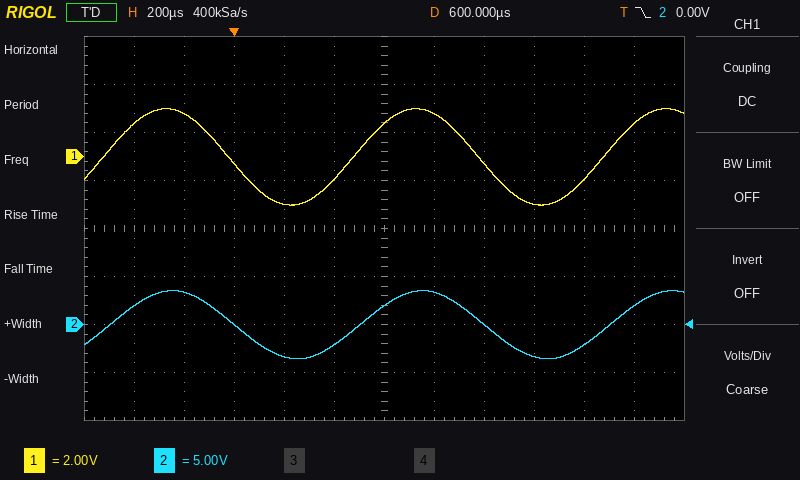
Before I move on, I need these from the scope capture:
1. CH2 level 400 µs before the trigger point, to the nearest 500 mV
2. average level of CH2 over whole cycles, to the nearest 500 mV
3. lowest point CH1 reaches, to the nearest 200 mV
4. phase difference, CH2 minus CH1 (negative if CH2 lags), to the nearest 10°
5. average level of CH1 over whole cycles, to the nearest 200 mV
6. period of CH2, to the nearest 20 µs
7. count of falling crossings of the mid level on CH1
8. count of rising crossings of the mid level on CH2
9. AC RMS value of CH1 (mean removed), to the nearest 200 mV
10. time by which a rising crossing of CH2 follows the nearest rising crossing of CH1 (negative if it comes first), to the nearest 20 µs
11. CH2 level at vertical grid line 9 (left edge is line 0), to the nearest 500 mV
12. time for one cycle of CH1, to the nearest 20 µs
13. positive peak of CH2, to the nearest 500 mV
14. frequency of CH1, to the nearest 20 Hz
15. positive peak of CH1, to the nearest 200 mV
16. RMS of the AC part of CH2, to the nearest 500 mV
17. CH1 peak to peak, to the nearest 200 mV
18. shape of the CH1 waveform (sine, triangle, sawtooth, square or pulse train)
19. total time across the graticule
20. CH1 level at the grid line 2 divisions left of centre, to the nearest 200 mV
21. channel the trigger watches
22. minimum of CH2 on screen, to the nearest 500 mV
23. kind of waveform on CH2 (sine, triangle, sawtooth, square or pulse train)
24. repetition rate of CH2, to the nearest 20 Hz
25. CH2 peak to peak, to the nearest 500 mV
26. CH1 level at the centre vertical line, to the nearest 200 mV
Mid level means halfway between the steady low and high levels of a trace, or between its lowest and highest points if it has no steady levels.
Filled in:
2.0 V
0.0 V
-2.0 V
-10°
0.0 V
1.00 ms
2
3
1.4 V
+20 µs
-3.5 V
1.00 ms
3.5 V
1.00 kHz
2.0 V
2.5 V
4.0 V
sine
2.4 ms
-2.0 V
CH2
-3.5 V
sine
1.00 kHz
7.0 V
1.4 V
